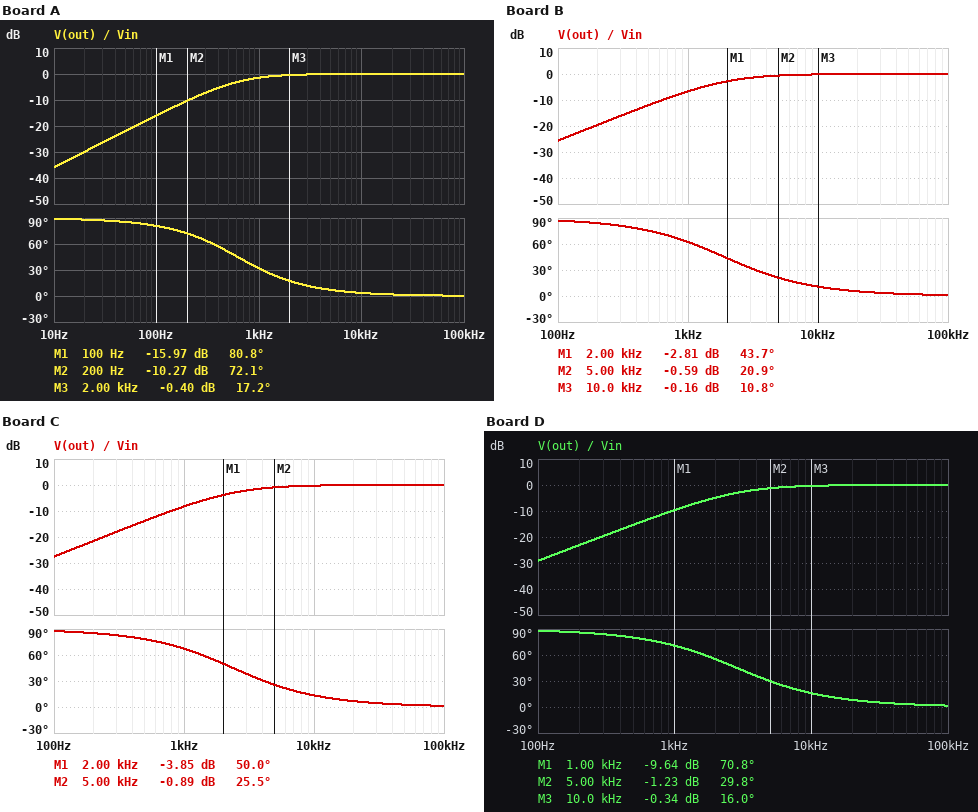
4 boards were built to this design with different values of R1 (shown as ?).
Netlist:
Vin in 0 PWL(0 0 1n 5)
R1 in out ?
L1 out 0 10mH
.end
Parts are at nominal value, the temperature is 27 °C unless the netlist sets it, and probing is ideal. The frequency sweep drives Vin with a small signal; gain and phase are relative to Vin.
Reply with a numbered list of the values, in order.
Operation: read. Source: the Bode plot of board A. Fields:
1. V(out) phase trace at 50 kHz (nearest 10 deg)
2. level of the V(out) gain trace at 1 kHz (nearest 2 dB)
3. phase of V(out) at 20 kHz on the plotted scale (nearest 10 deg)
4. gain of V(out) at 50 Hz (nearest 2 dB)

1. 0 deg
2. -2 dB
3. 0 deg
4. -22 dB
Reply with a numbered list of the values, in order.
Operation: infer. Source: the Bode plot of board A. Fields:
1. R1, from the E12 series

1. 39 Ω
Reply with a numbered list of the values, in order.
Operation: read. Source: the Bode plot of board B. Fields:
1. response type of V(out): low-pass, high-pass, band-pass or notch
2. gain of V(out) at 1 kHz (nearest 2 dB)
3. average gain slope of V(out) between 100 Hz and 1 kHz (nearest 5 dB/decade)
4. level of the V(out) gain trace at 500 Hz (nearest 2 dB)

1. high-pass
2. -6 dB
3. 20 dB/decade
4. -12 dB
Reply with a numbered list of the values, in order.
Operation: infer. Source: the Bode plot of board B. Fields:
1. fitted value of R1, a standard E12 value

1. 120 Ω
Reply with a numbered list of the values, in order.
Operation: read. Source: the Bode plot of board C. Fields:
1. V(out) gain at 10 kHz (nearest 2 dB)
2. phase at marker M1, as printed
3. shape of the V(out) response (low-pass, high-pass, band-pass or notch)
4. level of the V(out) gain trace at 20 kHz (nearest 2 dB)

1. 0 dB
2. 50.0 deg
3. high-pass
4. 0 dB
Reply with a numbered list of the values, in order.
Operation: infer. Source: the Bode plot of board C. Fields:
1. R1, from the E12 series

1. 150 Ω
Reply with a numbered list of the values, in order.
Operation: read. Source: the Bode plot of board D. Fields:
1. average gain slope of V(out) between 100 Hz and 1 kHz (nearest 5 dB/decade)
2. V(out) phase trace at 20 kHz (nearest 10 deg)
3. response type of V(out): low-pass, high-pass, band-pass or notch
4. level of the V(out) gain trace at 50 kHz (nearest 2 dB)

1. 20 dB/decade
2. 10 deg
3. high-pass
4. 0 dB
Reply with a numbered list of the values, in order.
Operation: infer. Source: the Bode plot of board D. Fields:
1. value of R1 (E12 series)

1. 180 Ω
